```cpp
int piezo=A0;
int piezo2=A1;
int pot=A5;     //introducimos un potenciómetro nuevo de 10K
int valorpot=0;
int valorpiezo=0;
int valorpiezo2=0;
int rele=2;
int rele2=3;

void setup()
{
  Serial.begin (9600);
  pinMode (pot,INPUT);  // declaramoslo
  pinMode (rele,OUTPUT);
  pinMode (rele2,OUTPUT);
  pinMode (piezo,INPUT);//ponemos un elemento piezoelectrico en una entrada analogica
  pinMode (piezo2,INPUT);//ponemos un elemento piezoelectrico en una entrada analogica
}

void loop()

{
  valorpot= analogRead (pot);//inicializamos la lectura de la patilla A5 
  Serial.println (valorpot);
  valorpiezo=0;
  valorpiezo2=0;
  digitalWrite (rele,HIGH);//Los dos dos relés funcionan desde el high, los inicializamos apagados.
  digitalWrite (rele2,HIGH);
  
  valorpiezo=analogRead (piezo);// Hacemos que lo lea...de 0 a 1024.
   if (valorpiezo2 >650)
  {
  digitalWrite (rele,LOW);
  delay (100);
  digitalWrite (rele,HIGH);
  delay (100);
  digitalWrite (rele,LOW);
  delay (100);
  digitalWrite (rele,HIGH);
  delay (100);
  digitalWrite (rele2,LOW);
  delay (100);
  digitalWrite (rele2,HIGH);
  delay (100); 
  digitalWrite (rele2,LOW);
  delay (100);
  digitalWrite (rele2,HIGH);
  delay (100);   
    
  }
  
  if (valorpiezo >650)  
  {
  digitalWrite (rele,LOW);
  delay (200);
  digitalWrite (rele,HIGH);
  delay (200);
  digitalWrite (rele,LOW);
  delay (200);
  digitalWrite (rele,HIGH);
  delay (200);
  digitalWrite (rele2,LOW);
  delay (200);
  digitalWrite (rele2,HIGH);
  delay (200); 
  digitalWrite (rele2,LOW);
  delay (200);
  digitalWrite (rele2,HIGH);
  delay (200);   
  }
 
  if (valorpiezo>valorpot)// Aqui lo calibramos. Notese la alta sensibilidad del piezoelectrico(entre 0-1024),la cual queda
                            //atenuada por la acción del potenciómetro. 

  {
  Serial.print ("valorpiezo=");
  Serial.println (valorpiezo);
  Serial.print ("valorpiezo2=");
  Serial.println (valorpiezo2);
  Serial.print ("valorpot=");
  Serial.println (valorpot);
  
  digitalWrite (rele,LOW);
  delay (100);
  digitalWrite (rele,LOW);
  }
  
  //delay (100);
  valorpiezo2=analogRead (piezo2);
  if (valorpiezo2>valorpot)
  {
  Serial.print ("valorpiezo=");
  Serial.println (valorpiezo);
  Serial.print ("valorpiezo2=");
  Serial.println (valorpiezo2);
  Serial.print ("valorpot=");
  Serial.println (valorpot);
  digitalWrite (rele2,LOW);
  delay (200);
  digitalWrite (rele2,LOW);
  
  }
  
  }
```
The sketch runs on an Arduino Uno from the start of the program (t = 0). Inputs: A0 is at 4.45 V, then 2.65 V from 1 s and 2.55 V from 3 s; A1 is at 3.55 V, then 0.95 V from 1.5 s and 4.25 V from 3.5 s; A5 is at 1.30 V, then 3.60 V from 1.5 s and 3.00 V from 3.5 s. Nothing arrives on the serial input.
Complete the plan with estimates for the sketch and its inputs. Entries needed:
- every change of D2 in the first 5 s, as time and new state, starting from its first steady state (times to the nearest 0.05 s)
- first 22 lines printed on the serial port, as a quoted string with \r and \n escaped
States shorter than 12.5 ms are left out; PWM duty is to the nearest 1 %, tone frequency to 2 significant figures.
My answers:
0 s low; 0.2 s high; 0.4 s low; 0.6 s high; 1.6 s low; 1.7 s high
"266\r\nvalorpiezo=911\r\nvalorpiezo2=0\r\nvalorpot=266\r\n737\r\n737\r\n737\r\n737\r\n737\r\n737\r\n737\r\n737\r\n737\r\n737\r\n737\r\n737\r\n737\r\n737\r\n737\r\n737\r\n737\r\n737\r\n"
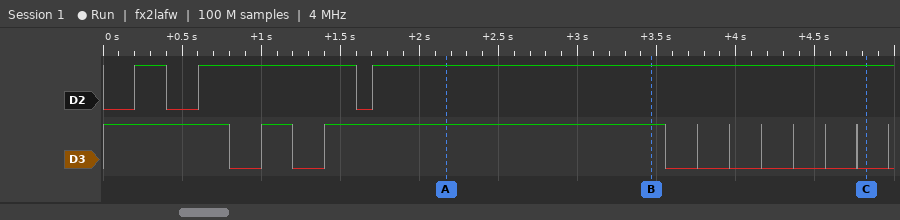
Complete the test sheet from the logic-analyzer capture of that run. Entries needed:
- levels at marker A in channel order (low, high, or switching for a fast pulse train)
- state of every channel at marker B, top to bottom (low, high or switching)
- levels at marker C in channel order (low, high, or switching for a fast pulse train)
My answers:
D2 high, D3 high
D2 high, D3 high
D2 high, D3 low
